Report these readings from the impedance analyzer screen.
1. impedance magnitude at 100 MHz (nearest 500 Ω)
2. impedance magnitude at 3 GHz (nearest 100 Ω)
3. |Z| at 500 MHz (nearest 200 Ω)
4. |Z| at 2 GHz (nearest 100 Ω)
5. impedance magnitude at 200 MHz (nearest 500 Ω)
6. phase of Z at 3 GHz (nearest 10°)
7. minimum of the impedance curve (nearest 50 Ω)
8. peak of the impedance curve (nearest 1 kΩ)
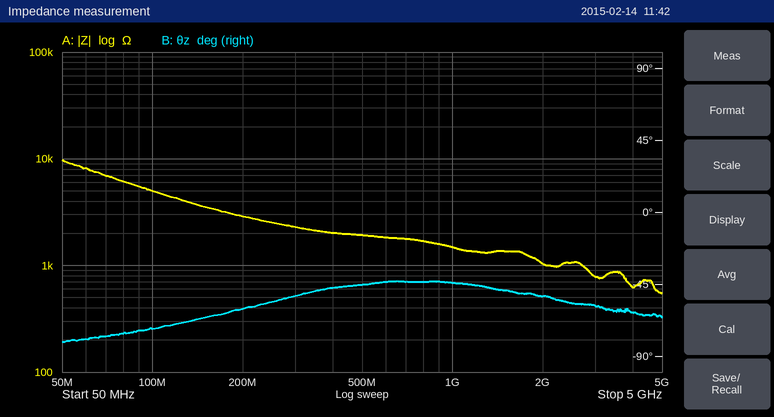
5.0 kΩ
800 Ω
2.0 kΩ
1.0 kΩ
3.0 kΩ
-60°
550 Ω
10 kΩ
